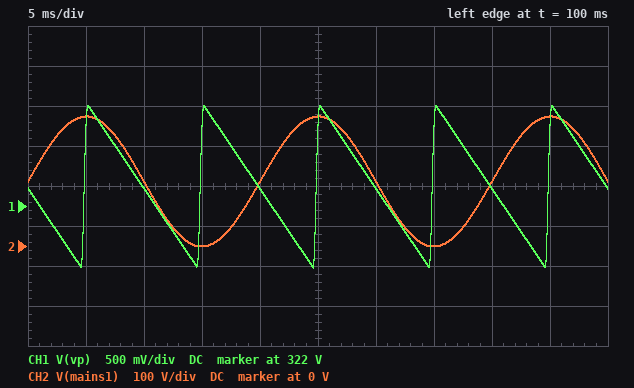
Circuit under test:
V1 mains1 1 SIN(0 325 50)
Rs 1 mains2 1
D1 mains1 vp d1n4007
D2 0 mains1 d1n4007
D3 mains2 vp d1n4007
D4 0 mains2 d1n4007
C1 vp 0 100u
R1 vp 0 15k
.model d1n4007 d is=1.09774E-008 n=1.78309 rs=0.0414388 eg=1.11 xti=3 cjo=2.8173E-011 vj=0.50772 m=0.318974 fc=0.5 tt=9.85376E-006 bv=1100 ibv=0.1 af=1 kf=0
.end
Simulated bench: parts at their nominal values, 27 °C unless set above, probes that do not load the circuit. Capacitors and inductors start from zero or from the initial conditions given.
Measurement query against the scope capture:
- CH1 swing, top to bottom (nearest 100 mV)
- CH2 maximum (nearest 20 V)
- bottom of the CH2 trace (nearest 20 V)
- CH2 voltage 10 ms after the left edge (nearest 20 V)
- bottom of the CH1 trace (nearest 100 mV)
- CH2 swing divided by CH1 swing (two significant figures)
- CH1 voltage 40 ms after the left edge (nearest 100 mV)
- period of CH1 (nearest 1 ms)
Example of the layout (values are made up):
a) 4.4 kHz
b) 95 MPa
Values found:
a) 2.0 V
b) 320 V
c) 0 V
d) 160 V
e) 321.2 V
f) 160
g) 322.2 V
h) 10 ms
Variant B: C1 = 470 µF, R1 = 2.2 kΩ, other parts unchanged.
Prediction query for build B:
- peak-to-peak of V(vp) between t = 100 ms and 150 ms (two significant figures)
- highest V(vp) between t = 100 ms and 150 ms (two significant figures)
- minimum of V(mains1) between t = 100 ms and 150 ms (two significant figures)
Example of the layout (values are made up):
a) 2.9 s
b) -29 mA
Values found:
a) 2.8 V
b) 320 V
c) -990 mV
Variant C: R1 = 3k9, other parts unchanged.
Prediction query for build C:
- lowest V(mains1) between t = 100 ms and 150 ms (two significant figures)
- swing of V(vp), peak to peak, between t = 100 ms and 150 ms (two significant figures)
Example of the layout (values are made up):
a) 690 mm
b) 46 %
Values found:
a) -930 mV
b) 7.5 V
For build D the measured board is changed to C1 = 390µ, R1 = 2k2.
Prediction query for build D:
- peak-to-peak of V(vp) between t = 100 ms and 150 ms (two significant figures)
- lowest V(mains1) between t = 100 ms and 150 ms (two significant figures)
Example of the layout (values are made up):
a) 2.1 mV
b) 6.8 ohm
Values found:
a) 3.4 V
b) -990 mV
